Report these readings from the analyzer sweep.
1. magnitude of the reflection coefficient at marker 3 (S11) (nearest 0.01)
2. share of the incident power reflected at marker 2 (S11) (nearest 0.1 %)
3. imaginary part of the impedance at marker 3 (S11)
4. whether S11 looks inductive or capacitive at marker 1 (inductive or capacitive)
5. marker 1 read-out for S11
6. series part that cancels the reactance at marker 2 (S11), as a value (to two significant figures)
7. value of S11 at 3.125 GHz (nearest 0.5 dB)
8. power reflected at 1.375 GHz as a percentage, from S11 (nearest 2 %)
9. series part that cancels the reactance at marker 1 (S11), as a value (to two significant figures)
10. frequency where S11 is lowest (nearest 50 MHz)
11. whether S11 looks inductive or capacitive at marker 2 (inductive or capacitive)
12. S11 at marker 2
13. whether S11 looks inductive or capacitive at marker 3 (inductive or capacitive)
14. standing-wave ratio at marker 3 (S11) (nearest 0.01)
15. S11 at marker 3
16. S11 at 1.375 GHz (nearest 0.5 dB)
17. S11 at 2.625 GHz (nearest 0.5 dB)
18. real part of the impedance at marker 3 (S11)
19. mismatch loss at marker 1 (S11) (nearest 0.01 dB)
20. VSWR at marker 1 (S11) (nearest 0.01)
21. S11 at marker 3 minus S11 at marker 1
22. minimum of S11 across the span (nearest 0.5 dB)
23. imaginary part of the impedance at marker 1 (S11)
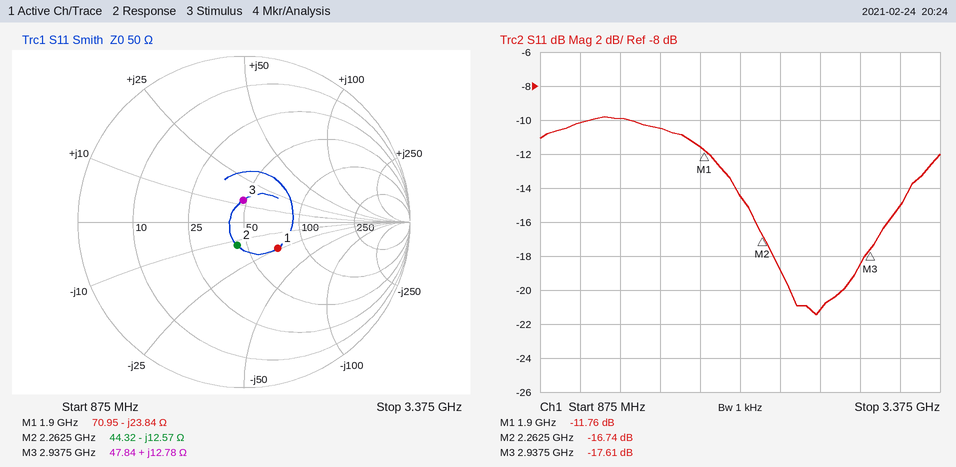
0.13
2.1 %
+12.78 Ω
capacitive
-11.76 dB
880 pH
-15.0 dB
10 %
2.0 nH
2.60 GHz
capacitive
-16.74 dB
inductive
1.30
-17.61 dB
-10.0 dB
-21.0 dB
47.84 Ω
0.30 dB
1.69
-5.85 dB
-21.5 dB
-23.84 Ω
